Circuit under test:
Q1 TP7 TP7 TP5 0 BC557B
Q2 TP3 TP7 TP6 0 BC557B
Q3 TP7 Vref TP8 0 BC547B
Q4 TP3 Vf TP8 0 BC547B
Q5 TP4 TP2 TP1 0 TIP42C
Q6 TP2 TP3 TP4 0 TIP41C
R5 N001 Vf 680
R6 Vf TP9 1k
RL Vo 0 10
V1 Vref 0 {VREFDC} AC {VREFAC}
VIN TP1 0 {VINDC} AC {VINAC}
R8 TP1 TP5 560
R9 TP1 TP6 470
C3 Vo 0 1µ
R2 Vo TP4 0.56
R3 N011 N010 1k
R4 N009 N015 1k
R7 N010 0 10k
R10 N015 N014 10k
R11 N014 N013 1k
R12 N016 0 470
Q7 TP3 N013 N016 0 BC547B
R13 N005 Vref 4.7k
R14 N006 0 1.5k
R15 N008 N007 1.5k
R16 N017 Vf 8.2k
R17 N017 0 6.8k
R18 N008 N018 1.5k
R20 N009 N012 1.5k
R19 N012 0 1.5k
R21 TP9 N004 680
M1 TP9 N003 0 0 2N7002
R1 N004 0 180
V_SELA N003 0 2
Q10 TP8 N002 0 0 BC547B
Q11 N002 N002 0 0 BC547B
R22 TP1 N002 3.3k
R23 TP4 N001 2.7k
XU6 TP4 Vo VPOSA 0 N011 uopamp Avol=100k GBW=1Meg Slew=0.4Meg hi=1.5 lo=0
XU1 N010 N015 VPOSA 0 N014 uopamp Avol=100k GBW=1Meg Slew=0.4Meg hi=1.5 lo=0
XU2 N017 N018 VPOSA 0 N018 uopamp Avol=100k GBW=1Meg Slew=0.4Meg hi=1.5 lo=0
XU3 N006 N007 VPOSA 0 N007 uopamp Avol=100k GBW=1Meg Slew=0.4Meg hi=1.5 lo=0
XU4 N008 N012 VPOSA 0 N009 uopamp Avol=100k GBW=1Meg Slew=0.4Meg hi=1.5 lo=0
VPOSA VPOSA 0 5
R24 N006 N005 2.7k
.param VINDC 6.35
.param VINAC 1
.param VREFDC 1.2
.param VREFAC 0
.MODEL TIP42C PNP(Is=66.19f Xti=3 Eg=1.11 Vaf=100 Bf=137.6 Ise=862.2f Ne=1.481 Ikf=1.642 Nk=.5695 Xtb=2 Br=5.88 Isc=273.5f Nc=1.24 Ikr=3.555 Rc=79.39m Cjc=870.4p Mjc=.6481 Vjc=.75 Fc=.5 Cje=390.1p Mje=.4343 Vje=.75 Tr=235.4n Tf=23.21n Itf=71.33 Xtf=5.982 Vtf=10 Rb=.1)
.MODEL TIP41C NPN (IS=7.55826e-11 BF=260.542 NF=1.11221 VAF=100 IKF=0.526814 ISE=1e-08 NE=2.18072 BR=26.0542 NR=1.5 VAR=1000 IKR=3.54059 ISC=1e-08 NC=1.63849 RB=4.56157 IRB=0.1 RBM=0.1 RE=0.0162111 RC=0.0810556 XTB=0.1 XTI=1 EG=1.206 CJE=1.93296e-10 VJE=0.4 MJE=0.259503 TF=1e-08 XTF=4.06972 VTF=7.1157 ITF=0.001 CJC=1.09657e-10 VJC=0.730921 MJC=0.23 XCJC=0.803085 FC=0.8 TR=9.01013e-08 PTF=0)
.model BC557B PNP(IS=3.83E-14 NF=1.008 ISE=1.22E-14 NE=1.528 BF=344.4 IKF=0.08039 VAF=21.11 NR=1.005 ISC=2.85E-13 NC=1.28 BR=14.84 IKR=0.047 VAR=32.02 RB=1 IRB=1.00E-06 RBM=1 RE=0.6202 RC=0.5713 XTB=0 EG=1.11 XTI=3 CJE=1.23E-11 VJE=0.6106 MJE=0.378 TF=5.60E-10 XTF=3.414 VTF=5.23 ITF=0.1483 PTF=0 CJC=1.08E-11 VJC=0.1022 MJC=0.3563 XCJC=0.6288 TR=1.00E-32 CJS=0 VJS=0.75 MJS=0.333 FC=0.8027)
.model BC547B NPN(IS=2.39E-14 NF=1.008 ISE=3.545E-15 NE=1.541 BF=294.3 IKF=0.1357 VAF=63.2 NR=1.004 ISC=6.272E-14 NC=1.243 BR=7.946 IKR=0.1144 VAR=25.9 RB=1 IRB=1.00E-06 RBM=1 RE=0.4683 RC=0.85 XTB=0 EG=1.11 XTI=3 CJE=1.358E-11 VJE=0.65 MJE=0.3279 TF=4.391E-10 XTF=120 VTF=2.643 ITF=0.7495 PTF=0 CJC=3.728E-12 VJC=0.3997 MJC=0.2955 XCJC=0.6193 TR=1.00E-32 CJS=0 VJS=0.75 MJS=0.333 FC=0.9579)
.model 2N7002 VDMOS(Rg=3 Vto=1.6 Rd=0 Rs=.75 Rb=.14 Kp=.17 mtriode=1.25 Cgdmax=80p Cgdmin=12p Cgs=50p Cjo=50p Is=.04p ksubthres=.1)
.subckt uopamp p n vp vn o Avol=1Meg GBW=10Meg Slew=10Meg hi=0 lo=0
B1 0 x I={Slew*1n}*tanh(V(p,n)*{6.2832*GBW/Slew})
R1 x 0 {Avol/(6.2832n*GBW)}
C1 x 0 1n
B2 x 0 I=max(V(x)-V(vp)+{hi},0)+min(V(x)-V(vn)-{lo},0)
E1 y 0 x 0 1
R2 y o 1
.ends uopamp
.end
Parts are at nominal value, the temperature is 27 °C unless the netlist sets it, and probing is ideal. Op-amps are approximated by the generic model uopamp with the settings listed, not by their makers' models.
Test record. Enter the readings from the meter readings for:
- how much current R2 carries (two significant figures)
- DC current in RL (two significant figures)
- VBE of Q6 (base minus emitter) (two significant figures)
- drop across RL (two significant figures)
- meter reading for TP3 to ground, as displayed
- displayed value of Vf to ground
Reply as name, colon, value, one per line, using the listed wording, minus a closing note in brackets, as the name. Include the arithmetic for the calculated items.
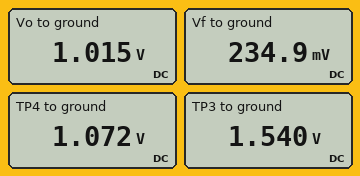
how much current R2 carries: (1.072 V - 1.015 V) / 560 mΩ = 100 mA
DC current in RL: (1.015 V) / 10 Ω = 100 mA
VBE of Q6 (base minus emitter): 1.54 V - 1.072 V = 470 mV
drop across RL: 1.015 V = 1.0 V
meter reading for TP3 to ground, as displayed: 1.540 V
displayed value of Vf to ground: 234.9 mV
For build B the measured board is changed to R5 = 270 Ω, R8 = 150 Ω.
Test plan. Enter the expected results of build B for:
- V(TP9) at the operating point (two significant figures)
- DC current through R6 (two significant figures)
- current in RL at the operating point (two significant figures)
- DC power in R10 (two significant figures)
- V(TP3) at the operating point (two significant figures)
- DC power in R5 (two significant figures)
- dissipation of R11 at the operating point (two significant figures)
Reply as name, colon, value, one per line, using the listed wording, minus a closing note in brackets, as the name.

V(TP9) at the operating point: 1.9 mV
DC current through R6: 150 µA
current in RL at the operating point: 60 mA
DC power in R10: 860 µW
V(TP3) at the operating point: 1.1 V
DC power in R5: 7.1 µW
dissipation of R11 at the operating point: 2.9 mW
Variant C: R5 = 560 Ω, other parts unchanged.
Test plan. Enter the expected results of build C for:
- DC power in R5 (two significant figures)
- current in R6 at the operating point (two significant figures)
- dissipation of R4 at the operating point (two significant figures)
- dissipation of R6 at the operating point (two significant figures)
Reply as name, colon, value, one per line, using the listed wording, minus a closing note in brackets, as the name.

DC power in R5: 36 µW
current in R6 at the operating point: 240 µA
dissipation of R4 at the operating point: 84 µW
dissipation of R6 at the operating point: 57 µW
